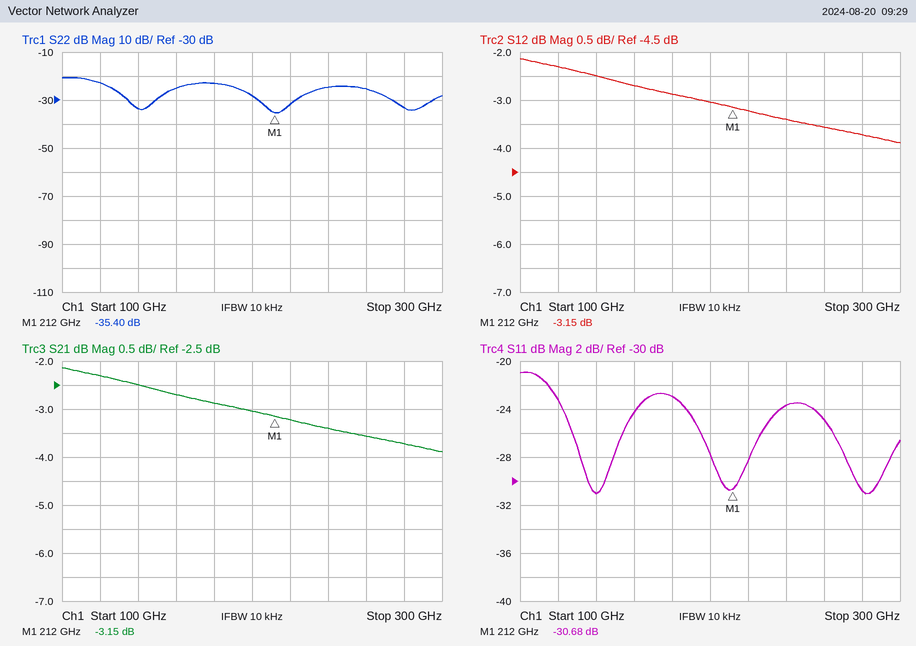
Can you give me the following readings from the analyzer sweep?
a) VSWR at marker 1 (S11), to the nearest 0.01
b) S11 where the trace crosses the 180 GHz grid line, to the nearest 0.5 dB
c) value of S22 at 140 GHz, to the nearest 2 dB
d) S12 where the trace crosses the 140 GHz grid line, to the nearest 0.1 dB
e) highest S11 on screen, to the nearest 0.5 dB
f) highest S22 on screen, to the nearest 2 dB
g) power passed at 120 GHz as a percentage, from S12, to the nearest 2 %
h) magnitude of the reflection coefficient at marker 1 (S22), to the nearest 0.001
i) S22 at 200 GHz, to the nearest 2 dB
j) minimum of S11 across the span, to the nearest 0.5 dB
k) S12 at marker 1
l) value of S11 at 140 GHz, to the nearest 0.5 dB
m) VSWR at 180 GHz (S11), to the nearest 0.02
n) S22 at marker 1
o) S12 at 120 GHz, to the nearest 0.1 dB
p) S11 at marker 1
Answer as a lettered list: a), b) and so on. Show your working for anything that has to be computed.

a) (1 + 0.0292)/(1 − 0.0292) ≈ 1.06
b) -23.0 dB
c) -34 dB
d) -2.5 dB
e) -21.0 dB
f) -20 dB
g) 10^(-2.3/10) ≈ 58.9 %, so 58 % to the nearest 2 %
h) 10^(-35.4/20) ≈ 0.017
i) -28 dB
j) -31.0 dB
k) -3.15 dB
l) -31.0 dB
m) |Γ| = 10^(-23/20) = 0.0708; VSWR = (1 + 0.0708)/(1 − 0.0708) ≈ 1.15, so 1.16 to the nearest 0.02
n) -35.40 dB
o) -2.3 dB
p) -30.68 dB
